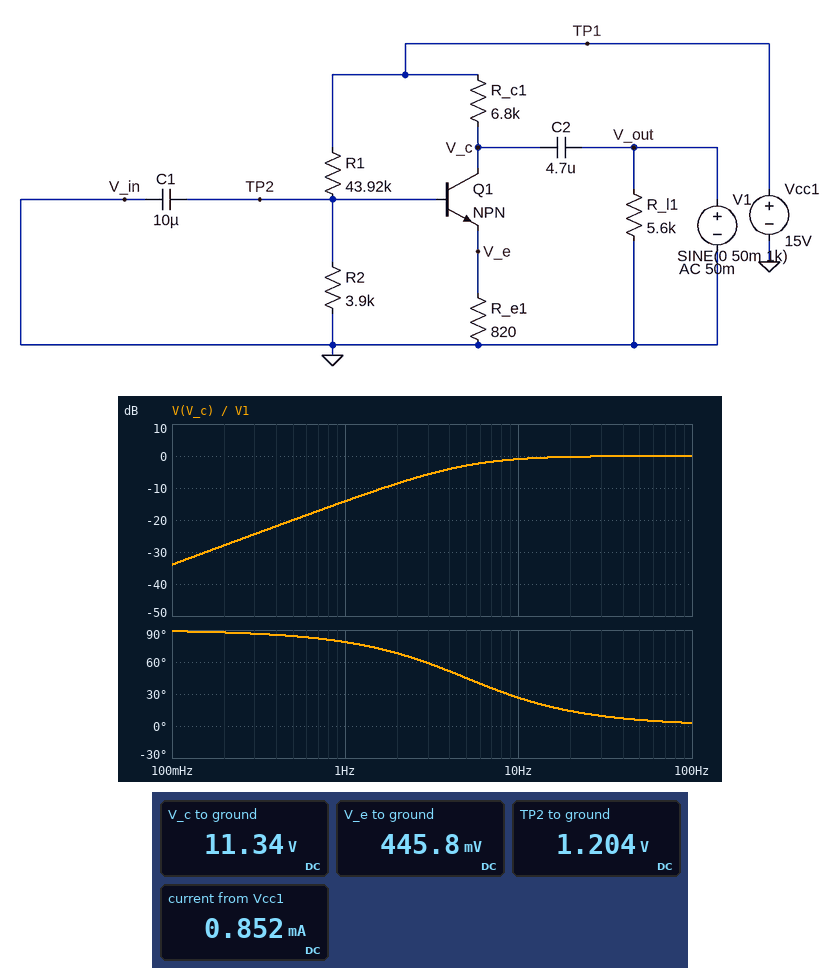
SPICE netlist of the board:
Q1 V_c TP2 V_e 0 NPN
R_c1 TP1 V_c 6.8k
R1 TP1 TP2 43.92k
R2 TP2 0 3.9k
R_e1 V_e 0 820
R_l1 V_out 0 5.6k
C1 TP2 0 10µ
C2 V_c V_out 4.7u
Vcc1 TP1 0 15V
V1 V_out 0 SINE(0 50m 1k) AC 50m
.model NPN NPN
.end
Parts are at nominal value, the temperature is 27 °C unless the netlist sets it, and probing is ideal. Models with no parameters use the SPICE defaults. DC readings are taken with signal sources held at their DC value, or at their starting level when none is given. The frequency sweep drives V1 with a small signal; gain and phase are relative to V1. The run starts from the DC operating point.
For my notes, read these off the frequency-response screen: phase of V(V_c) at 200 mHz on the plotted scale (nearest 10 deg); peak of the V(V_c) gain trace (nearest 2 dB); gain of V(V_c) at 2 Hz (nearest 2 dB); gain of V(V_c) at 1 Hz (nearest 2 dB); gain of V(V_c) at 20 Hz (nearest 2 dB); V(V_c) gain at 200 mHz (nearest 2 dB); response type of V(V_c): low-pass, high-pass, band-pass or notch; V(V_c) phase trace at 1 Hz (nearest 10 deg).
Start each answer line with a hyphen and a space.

- 90 deg
- 0 dB
- -8 dB
- -14 dB
- 0 dB
- -28 dB
- high-pass
- 80 deg
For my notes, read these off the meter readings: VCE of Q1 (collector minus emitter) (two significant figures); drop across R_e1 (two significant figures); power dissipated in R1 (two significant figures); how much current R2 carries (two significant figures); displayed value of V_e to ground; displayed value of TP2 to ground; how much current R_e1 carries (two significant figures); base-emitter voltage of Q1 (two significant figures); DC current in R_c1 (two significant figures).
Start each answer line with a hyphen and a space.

- 11 V
- 450 mV
- 4.3 mW
- 310 µA
- 445.8 mV
- 1.204 V
- 540 µA
- 760 mV
- 540 µA
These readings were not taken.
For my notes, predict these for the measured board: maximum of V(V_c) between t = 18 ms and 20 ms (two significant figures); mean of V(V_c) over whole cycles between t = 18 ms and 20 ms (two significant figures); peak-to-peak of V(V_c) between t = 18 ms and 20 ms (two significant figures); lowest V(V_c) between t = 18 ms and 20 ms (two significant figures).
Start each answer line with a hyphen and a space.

- 11 V
- 11 V
- 100 mV
- 11 V
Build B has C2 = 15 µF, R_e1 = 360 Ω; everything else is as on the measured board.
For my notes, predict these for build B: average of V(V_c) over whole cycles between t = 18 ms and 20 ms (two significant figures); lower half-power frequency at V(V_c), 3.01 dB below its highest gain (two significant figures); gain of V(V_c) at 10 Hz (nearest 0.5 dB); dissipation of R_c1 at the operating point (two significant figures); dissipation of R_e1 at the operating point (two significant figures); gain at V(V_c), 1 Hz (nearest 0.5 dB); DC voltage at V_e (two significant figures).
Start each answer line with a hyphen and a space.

- 7.4 V
- 1.6 Hz
- 0 dB
- 8.5 mW
- 460 µW
- -5.5 dB
- 410 mV
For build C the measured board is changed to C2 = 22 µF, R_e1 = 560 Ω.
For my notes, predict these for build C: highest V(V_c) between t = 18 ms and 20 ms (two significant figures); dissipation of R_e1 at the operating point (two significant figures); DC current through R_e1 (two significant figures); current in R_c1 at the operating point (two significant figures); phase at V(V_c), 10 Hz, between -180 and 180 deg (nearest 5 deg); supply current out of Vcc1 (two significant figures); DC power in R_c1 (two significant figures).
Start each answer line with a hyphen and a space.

- 9.9 V
- 330 µW
- 770 µA
- 760 µA
- 5 deg
- 1.1 mA
- 3.9 mW
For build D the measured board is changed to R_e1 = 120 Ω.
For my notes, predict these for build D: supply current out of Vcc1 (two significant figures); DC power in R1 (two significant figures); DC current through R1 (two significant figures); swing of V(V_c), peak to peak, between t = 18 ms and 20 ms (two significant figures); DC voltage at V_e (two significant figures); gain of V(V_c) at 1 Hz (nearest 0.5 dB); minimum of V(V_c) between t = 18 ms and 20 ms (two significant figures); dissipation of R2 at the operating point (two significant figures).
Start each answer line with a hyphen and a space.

- 2.5 mA
- 4.4 mW
- 320 µA
- 100 mV
- 260 mV
- -46.0 dB
- 350 mV
- 290 µW
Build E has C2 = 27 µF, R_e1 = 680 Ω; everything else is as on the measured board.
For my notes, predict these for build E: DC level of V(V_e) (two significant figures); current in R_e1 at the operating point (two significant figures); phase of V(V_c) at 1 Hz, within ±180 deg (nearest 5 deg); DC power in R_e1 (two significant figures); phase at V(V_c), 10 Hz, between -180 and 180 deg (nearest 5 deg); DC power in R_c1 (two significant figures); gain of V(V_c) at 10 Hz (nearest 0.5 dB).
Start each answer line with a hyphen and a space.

- 440 mV
- 640 µA
- 40 deg
- 280 µW
- 5 deg
- 2.8 mW
- 0 dB
